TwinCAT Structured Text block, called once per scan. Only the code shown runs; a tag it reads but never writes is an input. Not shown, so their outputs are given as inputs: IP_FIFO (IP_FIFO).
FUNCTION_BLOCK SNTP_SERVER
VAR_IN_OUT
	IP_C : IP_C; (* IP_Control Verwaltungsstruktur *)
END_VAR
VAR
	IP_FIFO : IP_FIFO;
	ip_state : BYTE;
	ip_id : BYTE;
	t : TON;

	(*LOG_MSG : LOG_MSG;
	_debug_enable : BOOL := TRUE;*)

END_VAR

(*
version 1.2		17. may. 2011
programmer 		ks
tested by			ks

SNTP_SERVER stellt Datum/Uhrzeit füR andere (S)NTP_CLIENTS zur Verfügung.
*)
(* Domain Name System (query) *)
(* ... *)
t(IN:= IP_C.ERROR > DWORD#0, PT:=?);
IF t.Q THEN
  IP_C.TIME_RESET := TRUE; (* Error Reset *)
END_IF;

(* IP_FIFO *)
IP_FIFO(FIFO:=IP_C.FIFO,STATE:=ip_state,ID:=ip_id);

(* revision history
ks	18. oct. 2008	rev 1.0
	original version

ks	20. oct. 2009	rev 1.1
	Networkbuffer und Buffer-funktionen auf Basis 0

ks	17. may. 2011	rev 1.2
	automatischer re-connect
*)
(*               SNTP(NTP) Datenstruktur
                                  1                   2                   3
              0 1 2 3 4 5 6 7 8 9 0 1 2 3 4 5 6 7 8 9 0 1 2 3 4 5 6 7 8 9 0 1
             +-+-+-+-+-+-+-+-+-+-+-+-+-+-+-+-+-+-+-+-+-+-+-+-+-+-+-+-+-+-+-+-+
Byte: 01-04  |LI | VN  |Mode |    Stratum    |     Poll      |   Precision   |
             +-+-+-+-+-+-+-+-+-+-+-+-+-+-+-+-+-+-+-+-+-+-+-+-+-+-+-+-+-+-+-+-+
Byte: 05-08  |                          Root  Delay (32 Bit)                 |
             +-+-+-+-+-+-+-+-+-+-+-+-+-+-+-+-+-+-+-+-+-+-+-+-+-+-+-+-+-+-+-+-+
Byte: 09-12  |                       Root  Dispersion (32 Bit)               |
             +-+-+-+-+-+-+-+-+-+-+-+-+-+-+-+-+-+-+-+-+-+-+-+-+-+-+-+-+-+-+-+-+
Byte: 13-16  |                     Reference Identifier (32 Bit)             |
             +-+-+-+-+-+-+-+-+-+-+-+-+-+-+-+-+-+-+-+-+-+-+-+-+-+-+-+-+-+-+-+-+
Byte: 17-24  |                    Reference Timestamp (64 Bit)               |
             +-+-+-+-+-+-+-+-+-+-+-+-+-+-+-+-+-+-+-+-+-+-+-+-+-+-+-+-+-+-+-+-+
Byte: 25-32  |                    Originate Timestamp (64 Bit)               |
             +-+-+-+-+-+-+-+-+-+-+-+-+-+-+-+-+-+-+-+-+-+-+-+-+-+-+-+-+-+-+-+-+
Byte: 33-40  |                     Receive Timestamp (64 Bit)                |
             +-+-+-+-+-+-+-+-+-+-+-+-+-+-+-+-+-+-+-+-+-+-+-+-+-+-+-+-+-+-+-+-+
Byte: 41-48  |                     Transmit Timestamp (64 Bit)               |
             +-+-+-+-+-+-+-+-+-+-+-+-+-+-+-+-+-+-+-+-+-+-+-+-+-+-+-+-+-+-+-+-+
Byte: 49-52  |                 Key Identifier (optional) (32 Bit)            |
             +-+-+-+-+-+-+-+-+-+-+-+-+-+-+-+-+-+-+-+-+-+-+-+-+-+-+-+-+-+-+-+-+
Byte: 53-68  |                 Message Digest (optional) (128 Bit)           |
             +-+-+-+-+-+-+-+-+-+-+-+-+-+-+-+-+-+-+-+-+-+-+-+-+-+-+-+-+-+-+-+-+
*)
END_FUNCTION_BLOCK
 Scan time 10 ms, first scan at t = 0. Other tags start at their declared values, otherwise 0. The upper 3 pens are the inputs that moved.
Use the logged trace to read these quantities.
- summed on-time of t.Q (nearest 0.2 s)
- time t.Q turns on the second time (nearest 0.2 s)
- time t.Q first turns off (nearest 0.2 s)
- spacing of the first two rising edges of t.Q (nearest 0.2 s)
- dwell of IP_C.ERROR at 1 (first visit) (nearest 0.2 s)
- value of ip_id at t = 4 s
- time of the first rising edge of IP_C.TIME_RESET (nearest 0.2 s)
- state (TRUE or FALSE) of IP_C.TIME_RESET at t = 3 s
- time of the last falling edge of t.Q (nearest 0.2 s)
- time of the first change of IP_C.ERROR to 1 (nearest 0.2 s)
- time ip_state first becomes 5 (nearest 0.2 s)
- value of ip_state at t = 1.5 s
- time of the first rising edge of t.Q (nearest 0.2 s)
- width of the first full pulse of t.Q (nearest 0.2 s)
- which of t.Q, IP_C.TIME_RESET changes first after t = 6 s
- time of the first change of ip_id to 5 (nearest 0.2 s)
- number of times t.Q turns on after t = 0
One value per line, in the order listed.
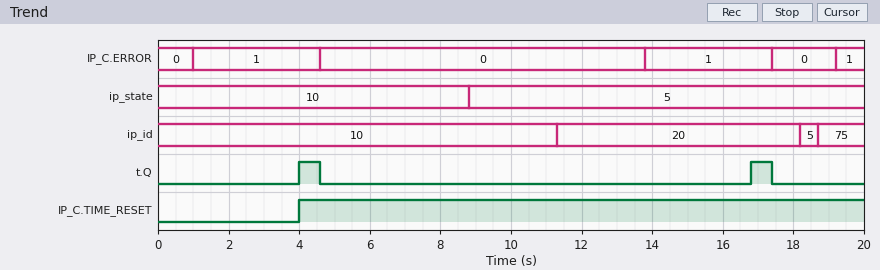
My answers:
1.2 s
16.8 s
4.6 s
12.8 s
3.6 s
10
4.0 s
FALSE
17.4 s
1.0 s
8.8 s
10
4.0 s
0.6 s
t.Q
18.2 s
2
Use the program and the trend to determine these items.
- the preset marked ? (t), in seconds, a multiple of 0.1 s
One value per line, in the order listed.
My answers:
3.0 s
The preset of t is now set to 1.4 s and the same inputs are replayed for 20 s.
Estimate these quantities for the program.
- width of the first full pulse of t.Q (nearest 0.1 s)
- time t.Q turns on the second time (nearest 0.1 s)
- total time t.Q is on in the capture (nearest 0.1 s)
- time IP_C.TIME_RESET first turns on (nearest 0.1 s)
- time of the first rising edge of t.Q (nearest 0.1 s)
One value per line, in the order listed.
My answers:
2.2 s
15.2 s
4.4 s
2.4 s
2.4 s
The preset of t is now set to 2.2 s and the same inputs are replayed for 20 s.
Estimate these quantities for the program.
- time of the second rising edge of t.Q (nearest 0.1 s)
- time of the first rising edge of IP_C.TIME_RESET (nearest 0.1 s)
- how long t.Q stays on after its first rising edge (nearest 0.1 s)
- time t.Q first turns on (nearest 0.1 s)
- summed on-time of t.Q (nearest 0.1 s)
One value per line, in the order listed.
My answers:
16.0 s
3.2 s
1.4 s
3.2 s
2.8 s
